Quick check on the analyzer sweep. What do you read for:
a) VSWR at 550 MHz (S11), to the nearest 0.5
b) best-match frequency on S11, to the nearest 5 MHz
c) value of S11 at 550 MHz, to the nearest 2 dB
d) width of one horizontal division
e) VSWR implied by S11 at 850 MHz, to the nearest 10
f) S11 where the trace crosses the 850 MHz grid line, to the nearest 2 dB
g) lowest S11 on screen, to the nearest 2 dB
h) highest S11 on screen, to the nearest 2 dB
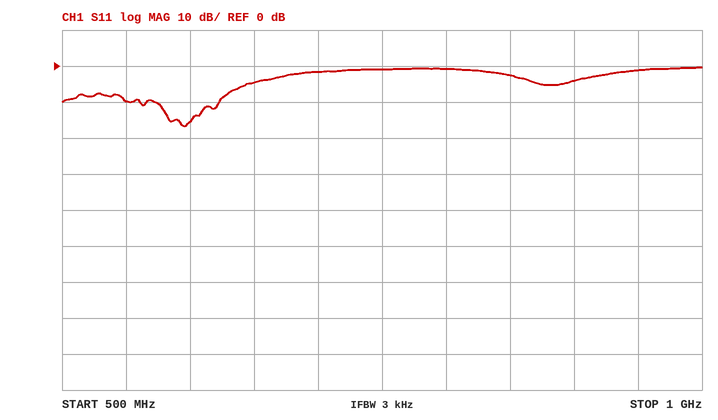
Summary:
2.0
595 MHz
-10 dB
50 MHz
10
-2 dB
-16 dB
0 dB
